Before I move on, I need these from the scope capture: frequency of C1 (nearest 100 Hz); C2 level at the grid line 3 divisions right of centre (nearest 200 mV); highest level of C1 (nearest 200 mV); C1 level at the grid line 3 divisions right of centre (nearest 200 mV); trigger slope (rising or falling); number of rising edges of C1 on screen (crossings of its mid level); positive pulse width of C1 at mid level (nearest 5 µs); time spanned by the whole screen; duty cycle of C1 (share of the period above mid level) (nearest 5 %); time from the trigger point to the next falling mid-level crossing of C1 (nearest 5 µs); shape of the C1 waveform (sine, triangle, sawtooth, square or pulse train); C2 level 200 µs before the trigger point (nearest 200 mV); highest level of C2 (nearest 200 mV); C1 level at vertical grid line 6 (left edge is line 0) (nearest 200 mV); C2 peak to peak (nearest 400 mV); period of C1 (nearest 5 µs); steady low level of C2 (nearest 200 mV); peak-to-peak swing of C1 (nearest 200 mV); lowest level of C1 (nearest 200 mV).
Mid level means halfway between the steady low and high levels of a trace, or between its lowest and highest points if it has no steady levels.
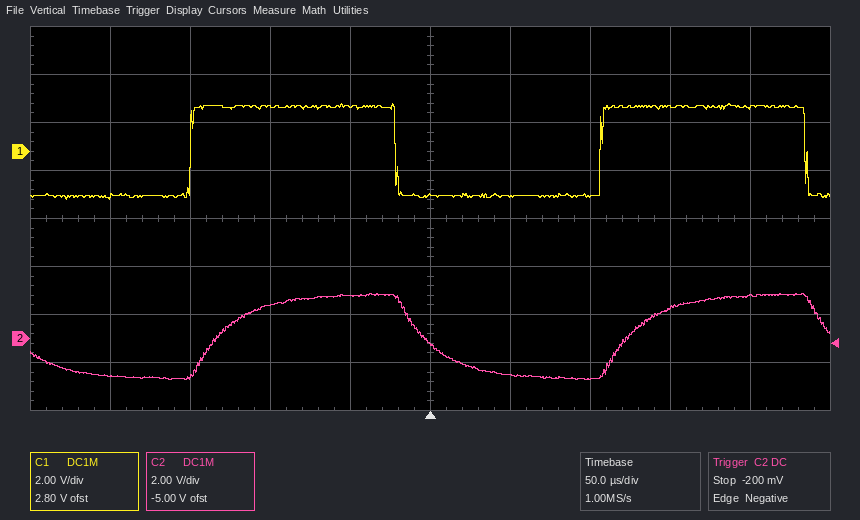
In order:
3.9 kHz
1.2 V
2.0 V
1.8 V
falling
2
130 µs
500 µs
50 %
235 µs
square
-1.6 V
1.8 V
-1.8 V
3.6 V
255 µs
-1.6 V
4.0 V
-2.0 V
